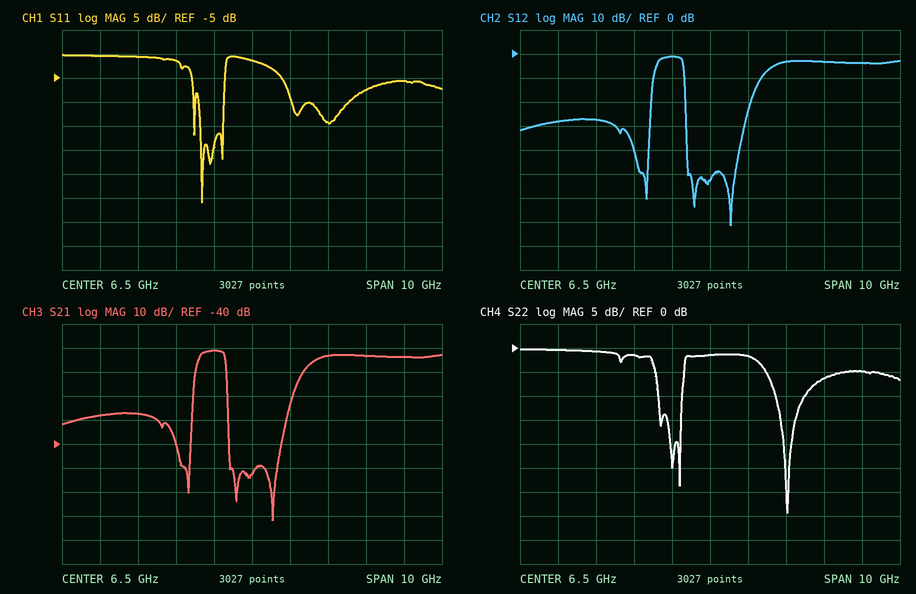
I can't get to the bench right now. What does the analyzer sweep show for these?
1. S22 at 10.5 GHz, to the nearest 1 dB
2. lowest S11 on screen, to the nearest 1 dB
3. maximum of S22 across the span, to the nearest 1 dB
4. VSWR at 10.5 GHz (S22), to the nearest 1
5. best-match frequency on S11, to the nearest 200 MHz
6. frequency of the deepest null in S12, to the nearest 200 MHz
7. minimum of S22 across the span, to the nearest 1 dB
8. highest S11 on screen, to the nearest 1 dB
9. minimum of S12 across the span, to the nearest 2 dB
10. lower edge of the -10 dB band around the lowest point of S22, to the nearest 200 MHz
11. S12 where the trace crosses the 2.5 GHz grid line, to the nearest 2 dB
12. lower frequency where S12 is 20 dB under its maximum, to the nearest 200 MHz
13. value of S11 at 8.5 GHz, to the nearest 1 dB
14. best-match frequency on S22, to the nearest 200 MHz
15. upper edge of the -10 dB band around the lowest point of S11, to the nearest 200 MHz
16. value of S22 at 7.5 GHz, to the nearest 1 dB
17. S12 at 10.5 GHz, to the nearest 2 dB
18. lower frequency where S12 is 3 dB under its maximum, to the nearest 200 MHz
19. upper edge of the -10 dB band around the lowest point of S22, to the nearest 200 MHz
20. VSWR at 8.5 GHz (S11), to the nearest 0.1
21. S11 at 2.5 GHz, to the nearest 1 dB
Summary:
-5 dB
-31 dB
0 dB
4
5.2 GHz
7.0 GHz
-34 dB
0 dB
-72 dB
8.2 GHz
-28 dB
5.0 GHz
-14 dB
8.6 GHz
5.8 GHz
-2 dB
-4 dB
5.2 GHz
9.0 GHz
1.5
0 dB
